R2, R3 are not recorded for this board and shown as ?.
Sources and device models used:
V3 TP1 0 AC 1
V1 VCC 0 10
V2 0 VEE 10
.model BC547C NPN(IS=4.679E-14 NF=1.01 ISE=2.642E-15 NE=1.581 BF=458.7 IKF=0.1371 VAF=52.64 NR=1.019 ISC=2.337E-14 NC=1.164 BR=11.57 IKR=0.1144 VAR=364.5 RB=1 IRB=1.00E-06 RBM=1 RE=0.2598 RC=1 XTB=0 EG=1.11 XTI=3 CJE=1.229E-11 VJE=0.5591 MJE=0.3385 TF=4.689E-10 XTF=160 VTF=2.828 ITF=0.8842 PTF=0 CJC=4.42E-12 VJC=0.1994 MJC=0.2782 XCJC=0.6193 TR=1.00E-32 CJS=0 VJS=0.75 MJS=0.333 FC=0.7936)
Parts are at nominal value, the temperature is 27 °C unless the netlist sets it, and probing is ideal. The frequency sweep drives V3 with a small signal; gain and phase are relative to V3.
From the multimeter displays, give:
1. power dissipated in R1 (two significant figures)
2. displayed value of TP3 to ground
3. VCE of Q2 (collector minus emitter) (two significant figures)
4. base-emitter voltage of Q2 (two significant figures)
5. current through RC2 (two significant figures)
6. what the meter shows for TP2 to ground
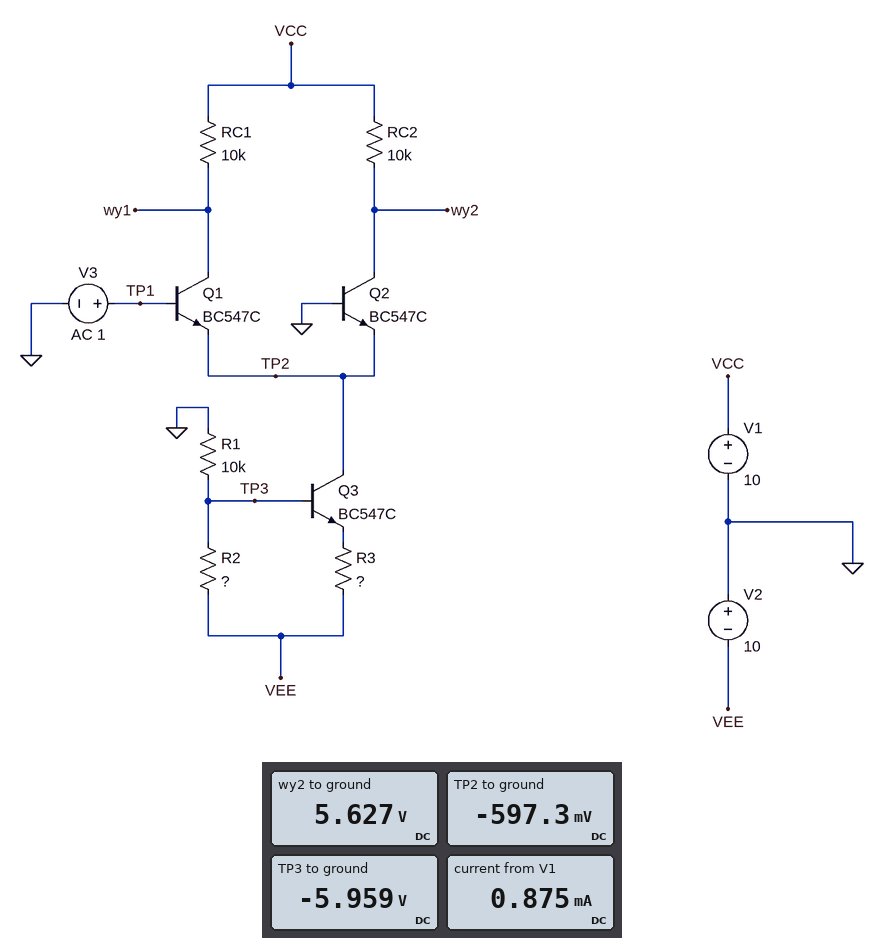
3.6 mW
-5.959 V
6.2 V
600 mV
440 µA
-597.3 mV
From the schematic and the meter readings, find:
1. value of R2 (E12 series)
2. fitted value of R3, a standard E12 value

6.8 kΩ
3.9 kΩ
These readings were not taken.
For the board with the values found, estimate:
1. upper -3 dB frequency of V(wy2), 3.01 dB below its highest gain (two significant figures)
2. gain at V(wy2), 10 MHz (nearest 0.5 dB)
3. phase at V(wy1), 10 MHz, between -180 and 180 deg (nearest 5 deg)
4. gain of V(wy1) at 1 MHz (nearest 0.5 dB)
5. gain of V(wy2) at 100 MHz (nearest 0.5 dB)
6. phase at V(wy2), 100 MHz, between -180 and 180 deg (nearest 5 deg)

9.7 MHz
34.5 dB
135 deg
37.5 dB
17.5 dB
-85 deg
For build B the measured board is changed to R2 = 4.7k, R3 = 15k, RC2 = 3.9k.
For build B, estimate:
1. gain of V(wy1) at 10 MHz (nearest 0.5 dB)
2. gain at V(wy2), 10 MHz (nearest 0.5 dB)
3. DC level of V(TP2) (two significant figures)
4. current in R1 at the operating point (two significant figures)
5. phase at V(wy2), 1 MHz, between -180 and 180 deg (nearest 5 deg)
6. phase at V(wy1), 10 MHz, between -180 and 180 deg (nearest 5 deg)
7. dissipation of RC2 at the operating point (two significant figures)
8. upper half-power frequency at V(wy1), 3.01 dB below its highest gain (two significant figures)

21.5 dB
15.5 dB
-550 mV
680 µA
0 deg
135 deg
30 µW
11 MHz
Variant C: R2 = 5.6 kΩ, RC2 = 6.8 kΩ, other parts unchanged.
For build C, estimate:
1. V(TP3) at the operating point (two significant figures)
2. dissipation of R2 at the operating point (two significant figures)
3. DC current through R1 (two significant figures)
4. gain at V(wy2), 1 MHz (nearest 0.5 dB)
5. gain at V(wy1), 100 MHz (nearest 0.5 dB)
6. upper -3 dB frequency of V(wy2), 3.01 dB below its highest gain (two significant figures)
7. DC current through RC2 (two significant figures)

-6.4 V
2.3 mW
640 µA
33.5 dB
16.5 dB
15 MHz
380 µA
